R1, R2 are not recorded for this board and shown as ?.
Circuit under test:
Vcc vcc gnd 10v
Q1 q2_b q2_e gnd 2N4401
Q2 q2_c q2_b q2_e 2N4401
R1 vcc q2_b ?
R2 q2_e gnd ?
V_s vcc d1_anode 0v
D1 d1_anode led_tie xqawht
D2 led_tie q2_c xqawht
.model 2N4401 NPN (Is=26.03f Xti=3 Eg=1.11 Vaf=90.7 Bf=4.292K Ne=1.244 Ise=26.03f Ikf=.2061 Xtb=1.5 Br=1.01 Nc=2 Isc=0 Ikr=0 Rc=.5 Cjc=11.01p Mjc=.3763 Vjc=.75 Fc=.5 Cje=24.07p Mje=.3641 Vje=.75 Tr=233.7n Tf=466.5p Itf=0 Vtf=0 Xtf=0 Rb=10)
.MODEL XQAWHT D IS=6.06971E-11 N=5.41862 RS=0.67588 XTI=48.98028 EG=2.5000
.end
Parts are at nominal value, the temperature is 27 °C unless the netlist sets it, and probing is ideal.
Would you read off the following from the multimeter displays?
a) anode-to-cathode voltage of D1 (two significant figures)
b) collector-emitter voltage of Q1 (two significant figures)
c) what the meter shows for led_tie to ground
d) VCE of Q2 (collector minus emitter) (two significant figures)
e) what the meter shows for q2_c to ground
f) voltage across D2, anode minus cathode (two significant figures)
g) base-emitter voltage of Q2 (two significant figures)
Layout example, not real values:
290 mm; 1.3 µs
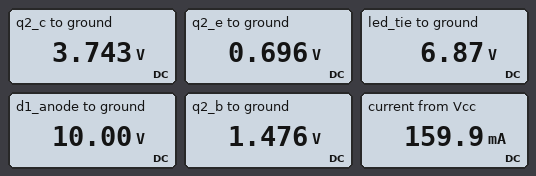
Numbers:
3.1 V; 1.5 V; 6.87 V; 3.0 V; 3.743 V; 3.1 V; 780 mV
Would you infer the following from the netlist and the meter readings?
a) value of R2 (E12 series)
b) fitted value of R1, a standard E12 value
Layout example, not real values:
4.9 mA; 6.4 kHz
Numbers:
4.7 Ω; 680 Ω
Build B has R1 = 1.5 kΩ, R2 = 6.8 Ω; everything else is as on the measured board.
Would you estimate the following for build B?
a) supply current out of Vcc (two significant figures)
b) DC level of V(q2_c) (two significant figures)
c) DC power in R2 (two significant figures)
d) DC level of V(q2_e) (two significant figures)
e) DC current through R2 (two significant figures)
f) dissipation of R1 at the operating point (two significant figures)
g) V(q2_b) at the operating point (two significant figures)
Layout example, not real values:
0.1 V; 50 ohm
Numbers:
100 mA; 3.9 V; 67 mW; 670 mV; 99 mA; 49 mW; 1.4 V
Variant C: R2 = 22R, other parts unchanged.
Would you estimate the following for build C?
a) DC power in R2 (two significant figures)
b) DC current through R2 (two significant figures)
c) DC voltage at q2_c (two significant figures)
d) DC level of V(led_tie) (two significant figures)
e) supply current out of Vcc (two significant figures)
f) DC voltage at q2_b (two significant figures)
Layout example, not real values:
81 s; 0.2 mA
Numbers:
22 mW; 32 mA; 4.3 V; 7.2 V; 44 mA; 1.4 V
